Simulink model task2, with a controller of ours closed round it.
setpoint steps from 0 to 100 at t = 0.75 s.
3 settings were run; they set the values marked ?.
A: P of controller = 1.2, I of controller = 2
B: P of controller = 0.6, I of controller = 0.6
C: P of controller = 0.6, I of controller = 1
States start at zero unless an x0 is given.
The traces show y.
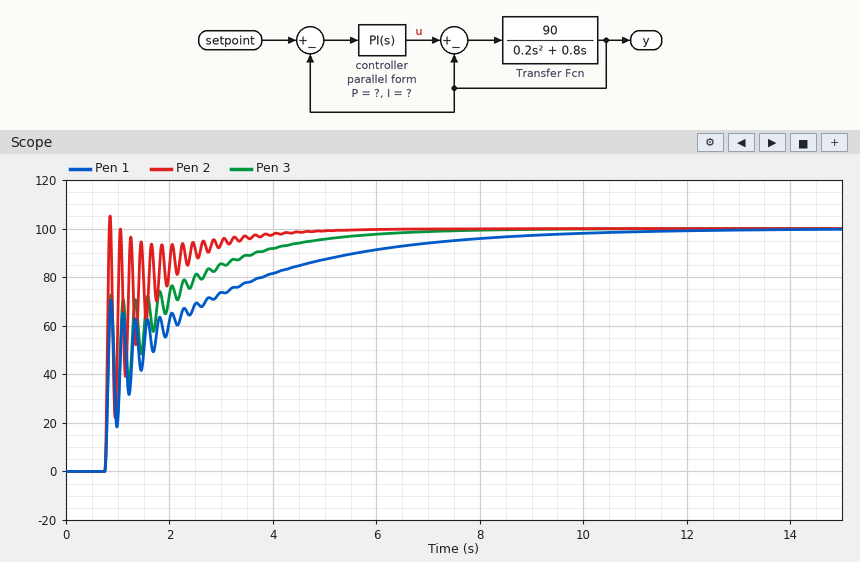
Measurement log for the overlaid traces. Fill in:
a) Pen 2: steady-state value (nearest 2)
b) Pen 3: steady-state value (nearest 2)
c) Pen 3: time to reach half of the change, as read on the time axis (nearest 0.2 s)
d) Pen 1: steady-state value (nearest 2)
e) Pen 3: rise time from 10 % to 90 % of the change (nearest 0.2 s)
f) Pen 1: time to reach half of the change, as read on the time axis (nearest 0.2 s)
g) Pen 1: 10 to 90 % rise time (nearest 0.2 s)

100
100
0.8 s
100
2.8 s
0.8 s
4.8 s
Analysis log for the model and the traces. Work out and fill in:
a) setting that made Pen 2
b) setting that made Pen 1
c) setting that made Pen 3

A
B
C
